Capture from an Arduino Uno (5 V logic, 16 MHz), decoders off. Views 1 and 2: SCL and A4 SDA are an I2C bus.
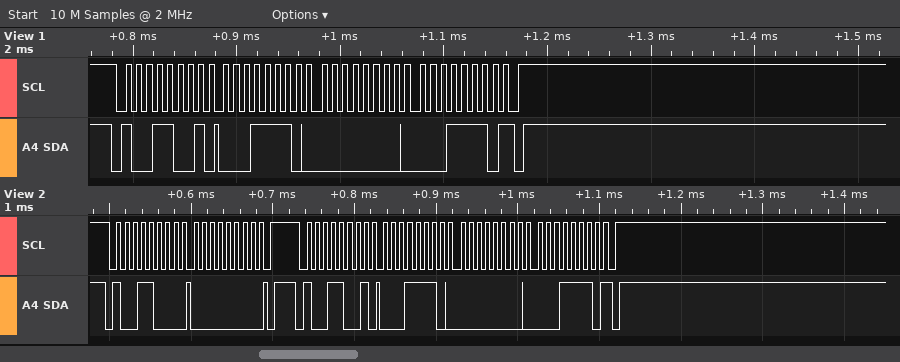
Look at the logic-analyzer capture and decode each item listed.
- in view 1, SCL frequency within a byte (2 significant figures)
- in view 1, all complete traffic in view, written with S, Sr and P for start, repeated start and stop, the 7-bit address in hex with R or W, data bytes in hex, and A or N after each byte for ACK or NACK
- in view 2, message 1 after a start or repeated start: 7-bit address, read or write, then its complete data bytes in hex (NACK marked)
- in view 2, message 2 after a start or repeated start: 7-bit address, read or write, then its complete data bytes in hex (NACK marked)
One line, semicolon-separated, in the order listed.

100 kHz; S 4CR A 1E A 00 A 1E N P; 0x4C write: 00; 0x4C read: 1E 00 1E NACK
